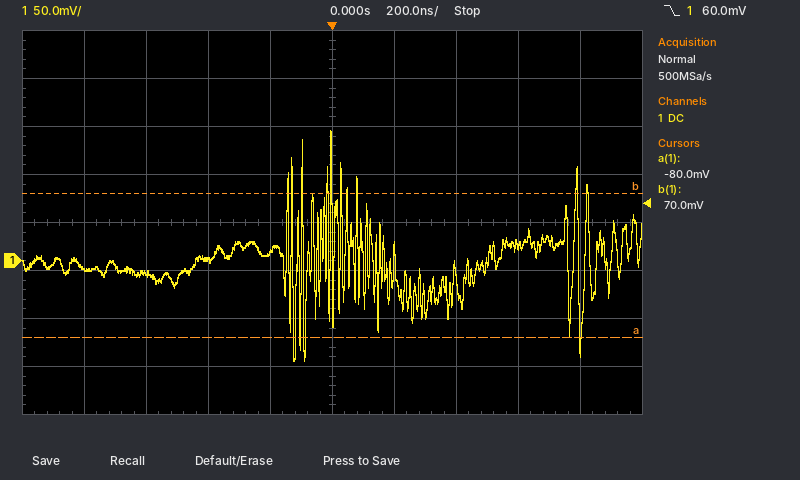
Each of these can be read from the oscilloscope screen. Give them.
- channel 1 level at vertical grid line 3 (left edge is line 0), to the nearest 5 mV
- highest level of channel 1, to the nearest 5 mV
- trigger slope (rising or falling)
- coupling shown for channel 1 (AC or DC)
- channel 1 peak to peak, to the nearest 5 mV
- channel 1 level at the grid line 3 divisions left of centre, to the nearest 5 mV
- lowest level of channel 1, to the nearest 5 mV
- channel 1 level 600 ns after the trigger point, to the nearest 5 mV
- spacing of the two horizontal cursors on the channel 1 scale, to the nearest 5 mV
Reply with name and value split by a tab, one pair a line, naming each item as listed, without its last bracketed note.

channel 1 level at vertical grid line 3 (left edge is line 0), to the nearest 5 mV	0 mV
highest level of channel 1, to the nearest 5 mV	135 mV
trigger slope	falling
coupling shown for channel 1	DC
channel 1 peak to peak, to the nearest 5 mV	240 mV
channel 1 level at the grid line 3 divisions left of centre, to the nearest 5 mV	-15 mV
lowest level of channel 1, to the nearest 5 mV	-105 mV
channel 1 level 600 ns after the trigger point, to the nearest 5 mV	15 mV
spacing of the two horizontal cursors on the channel 1 scale, to the nearest 5 mV	150 mV
